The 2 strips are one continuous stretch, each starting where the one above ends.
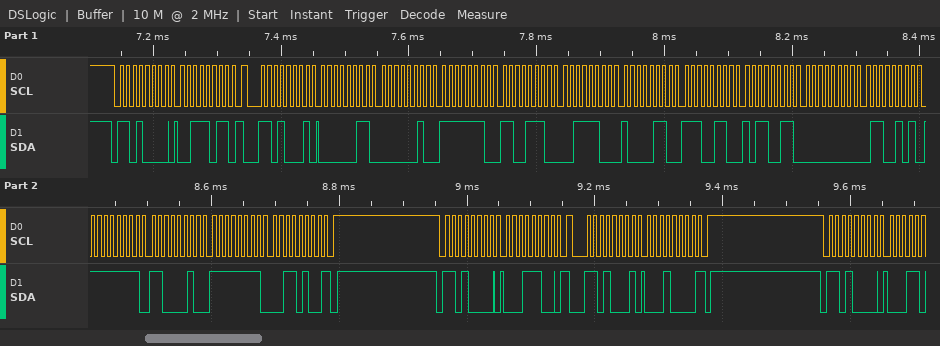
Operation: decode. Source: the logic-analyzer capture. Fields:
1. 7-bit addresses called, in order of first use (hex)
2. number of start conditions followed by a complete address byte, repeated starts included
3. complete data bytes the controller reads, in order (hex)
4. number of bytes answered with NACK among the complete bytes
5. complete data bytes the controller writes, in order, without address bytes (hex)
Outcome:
0x68
5
03 02 FE CE 3C 86 E6 B3 00 65 FF C2 FF 34 10
2
3B 1C
